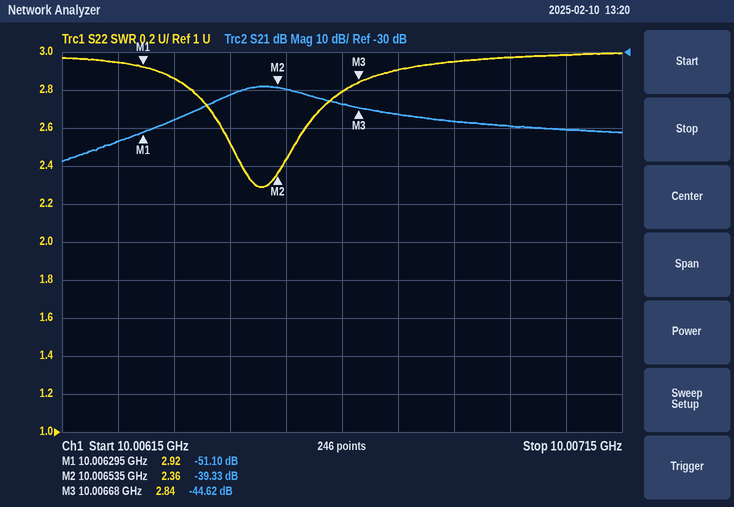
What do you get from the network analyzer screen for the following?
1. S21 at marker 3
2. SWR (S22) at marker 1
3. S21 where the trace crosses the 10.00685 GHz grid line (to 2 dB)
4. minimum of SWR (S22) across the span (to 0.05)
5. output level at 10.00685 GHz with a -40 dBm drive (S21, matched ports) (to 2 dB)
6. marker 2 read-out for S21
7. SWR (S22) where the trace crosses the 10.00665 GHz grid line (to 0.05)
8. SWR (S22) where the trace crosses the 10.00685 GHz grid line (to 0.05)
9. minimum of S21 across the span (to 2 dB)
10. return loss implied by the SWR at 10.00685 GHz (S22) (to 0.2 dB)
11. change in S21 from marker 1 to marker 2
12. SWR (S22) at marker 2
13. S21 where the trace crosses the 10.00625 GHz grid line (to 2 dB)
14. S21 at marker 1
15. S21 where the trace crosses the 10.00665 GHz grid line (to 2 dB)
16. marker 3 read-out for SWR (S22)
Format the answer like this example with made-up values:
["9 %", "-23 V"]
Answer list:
["-44.62 dB", "2.92", "-48 dB", "2.30", "-88 dBm", "-39.33 dB", "2.80", "2.95", "-58 dB", "6.2 dB", "11.77 dB", "2.36", "-54 dB", "-51.10 dB", "-44 dB", "2.84"]
